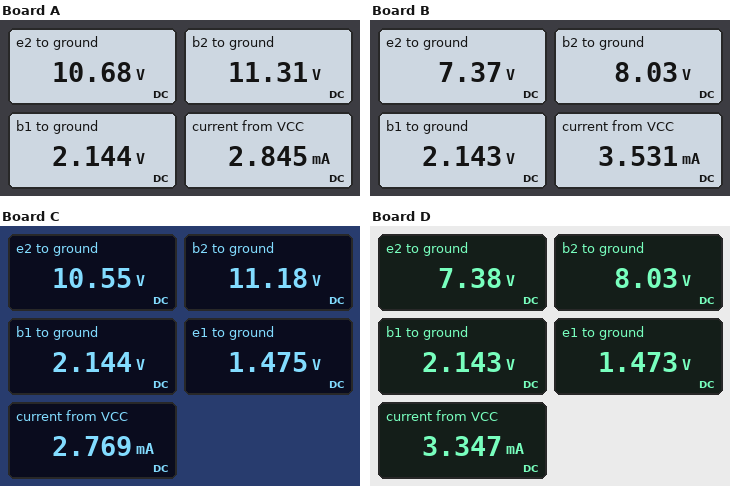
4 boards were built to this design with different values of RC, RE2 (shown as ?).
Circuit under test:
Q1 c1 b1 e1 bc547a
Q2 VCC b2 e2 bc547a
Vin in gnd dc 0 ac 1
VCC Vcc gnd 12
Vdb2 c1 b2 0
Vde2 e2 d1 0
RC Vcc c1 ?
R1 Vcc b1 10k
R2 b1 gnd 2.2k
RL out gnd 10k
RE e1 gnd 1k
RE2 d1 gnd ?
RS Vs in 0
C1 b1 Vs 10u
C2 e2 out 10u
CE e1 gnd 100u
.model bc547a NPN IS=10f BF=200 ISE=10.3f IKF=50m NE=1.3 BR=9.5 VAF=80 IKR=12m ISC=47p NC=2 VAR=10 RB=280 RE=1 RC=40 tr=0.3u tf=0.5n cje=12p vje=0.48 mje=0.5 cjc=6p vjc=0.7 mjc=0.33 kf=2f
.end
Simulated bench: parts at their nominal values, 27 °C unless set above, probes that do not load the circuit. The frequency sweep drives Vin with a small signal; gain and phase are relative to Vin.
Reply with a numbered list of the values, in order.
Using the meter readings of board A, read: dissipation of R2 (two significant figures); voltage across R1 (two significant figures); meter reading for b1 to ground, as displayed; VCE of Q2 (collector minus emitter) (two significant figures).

1. 2.1 mW
2. 9.9 V
3. 2.144 V
4. 1.3 V
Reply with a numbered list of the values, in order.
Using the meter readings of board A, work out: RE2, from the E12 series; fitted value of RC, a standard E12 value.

1. 27 kΩ
2. 470 Ω
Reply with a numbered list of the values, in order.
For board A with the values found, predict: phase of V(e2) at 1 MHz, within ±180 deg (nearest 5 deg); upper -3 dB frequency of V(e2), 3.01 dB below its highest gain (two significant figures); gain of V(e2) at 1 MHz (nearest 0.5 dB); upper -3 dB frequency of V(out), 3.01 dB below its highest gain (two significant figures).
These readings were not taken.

1. 165 deg
2. 4.7 MHz
3. 26.5 dB
4. 4.7 MHz
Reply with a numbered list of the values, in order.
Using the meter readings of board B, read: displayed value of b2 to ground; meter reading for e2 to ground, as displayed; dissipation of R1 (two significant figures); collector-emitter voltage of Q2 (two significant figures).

1. 8.03 V
2. 7.37 V
3. 9.7 mW
4. 4.6 V
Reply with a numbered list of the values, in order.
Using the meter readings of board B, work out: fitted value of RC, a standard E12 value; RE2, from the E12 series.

1. 2.7 kΩ
2. 6.8 kΩ
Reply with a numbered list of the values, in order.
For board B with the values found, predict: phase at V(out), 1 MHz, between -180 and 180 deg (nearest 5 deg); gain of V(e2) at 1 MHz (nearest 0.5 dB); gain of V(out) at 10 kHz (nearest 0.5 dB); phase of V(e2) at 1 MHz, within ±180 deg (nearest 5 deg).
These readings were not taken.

1. 140 deg
2. 39.5 dB
3. 41.5 dB
4. 140 deg
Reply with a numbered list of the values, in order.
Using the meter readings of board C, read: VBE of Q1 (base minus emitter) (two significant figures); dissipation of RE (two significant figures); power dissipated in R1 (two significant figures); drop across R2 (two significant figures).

1. 670 mV
2. 2.2 mW
3. 9.7 mW
4. 2.1 V
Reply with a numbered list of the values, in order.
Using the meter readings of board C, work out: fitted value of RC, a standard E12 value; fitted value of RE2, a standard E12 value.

1. 560 Ω
2. 33 kΩ
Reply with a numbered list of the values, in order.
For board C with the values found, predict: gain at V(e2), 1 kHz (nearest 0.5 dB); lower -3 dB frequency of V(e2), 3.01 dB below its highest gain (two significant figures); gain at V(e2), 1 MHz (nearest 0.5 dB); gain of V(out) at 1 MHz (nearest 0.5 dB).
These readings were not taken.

1. 28.0 dB
2. 83 Hz
3. 28.0 dB
4. 28.0 dB
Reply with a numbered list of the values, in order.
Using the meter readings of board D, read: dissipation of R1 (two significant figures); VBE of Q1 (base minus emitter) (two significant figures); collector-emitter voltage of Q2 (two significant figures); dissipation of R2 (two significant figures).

1. 9.7 mW
2. 670 mV
3. 4.6 V
4. 2.1 mW
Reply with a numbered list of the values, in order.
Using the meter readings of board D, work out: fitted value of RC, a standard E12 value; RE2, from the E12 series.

1. 2.7 kΩ
2. 8.2 kΩ
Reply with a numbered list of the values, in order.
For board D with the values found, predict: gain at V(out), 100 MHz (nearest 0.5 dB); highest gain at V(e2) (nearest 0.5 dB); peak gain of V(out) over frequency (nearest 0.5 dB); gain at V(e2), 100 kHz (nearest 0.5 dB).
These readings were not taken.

1. -2.5 dB
2. 41.5 dB
3. 41.5 dB
4. 41.5 dB
